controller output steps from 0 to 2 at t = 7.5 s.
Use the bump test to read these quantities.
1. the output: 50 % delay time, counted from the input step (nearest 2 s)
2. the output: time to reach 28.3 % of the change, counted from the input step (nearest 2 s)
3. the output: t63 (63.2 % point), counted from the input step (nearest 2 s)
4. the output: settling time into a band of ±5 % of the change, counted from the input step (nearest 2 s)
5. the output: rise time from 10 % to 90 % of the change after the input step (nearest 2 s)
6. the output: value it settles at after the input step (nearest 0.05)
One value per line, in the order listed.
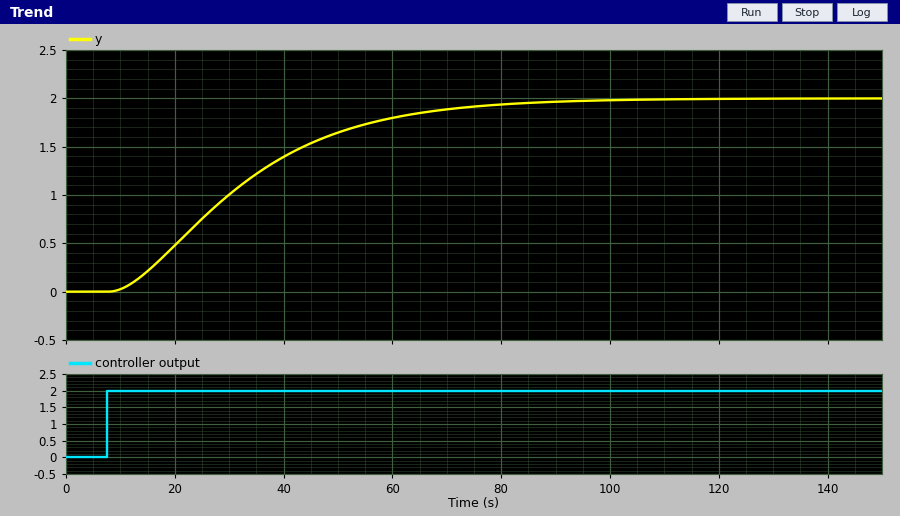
22 s
14 s
28 s
64 s
46 s
2.00
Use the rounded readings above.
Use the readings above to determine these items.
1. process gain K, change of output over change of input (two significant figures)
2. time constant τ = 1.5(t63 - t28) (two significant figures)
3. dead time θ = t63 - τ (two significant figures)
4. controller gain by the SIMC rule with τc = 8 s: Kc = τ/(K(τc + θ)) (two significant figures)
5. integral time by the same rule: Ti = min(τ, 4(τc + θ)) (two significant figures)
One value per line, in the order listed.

1.0
21 s
7.0 s
1.4
21 s
